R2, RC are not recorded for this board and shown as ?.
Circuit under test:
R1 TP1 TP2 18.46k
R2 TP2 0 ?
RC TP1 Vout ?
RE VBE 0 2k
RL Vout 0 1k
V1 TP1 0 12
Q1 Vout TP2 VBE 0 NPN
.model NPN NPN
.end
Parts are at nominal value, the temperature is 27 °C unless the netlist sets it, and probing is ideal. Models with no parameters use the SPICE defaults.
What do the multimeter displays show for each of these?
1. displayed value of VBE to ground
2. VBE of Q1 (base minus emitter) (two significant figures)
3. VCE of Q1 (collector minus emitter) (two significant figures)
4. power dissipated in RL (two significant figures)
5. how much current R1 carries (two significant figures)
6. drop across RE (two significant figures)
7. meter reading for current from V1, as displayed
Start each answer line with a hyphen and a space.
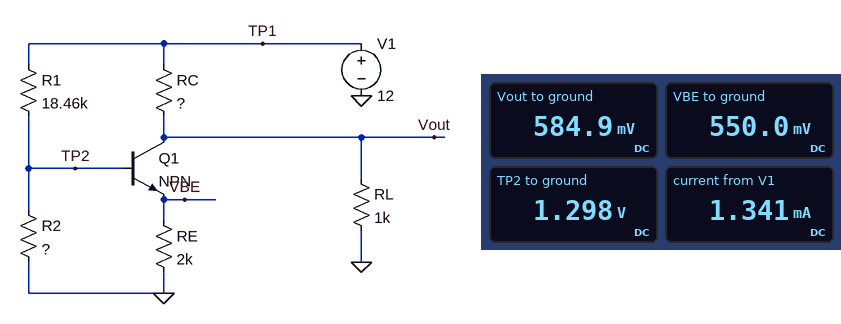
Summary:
- 550.0 mV
- 750 mV
- 35 mV
- 340 µW
- 580 µA
- 550 mV
- 1.341 mA
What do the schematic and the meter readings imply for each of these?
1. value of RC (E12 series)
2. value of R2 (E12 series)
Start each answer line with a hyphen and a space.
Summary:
- 15 kΩ
- 2.7 kΩ
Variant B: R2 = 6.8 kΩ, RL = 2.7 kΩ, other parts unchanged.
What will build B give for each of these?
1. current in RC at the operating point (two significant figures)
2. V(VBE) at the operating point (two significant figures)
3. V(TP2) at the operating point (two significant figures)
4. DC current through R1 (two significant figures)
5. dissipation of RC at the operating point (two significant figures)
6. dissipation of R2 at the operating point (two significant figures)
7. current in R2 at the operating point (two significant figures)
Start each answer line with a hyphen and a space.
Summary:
- 720 µA
- 1.1 V
- 1.9 V
- 550 µA
- 7.8 mW
- 530 µW
- 280 µA
